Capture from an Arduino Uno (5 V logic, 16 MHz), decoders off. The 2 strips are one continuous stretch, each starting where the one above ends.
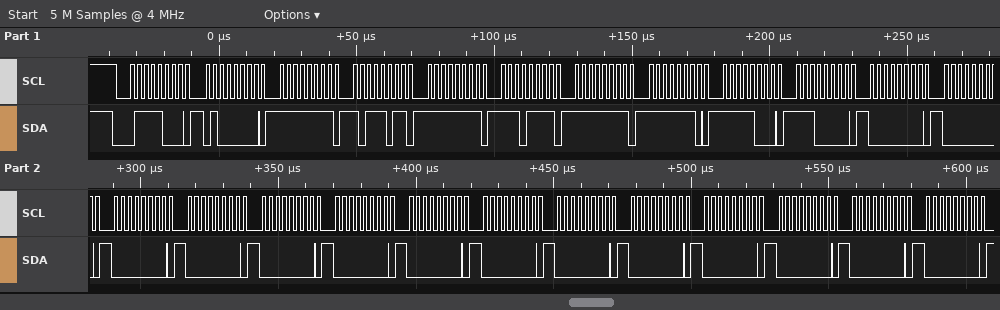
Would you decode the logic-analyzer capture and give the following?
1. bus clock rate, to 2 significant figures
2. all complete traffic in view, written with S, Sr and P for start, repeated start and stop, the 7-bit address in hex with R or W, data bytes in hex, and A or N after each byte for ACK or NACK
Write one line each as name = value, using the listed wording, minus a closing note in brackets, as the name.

bus clock rate, to 2 significant figures = 400 kHz
all complete traffic in view, written with S, Sr and P for start, repeated start and stop, the 7-bit address in hex with R or W, data bytes in hex, and A or N after each byte for ACK or NACK = S 3CW A 40 A FF A BB A FF A EF A FF A FE A F8 A E0 A 00 A 00 A 00 A 00 A 00 A 00 A 00 A 00 A 00 A 00 A 00 A 00 A 00 A 00 A
